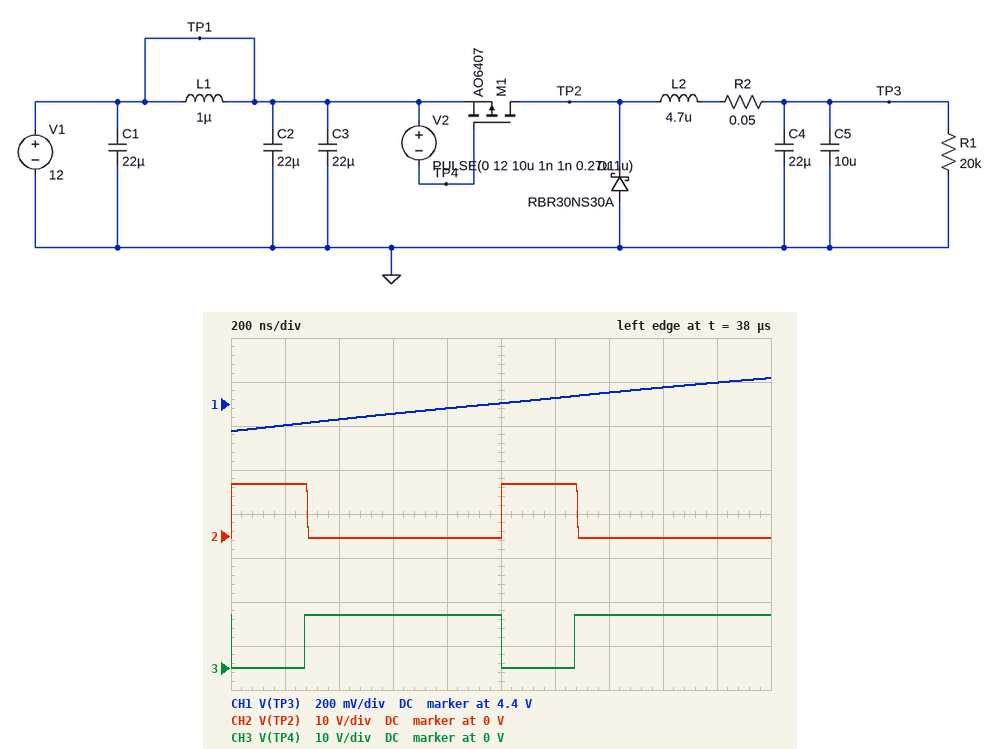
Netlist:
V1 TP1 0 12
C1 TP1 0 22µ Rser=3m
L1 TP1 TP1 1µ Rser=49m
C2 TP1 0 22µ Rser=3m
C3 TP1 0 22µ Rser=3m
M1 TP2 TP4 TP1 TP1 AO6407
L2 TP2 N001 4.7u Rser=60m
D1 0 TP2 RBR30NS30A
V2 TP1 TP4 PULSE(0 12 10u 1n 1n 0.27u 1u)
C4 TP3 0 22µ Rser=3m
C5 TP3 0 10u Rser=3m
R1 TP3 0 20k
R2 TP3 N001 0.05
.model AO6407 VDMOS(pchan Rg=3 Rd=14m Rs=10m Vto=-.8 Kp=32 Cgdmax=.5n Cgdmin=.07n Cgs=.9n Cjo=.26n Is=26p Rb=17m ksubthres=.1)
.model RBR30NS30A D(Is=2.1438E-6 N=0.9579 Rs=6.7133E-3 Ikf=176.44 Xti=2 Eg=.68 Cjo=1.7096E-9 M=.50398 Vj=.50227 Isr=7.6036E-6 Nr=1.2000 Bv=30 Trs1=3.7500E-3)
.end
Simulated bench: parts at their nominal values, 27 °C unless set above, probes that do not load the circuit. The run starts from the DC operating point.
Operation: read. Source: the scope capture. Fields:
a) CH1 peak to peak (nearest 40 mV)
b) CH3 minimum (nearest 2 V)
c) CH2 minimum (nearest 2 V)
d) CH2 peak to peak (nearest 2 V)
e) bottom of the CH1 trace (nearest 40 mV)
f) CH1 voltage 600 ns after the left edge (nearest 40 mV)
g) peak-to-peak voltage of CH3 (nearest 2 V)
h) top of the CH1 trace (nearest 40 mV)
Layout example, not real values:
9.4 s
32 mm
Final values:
240 mV
0 V
0 V
12 V
4.28 V
4.36 V
12 V
4.52 V
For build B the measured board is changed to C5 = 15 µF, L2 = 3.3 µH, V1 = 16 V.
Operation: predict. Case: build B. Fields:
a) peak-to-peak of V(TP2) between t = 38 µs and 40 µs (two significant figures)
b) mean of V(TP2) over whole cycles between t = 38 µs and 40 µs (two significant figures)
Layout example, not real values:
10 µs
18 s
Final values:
16 V
4.2 V
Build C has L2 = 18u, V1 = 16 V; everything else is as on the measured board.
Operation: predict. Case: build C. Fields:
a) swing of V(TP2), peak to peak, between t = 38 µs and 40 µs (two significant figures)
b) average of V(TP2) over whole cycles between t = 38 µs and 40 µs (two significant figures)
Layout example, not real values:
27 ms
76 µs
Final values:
16 V
4.2 V
